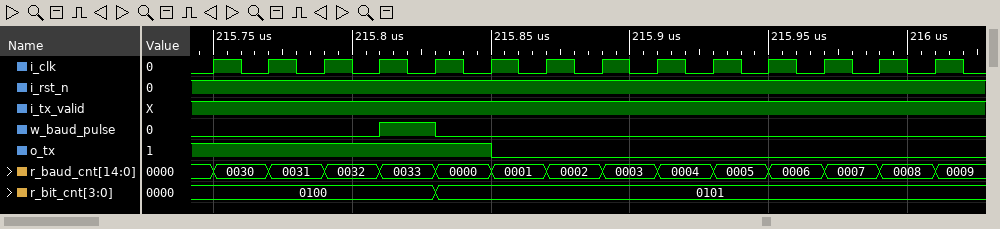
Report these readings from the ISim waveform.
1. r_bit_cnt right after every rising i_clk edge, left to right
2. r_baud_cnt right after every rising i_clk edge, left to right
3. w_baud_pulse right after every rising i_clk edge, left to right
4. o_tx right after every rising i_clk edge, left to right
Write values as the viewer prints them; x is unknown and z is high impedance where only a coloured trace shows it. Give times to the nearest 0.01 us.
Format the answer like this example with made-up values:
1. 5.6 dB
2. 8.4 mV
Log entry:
1. 0100, 0100, 0100, 0100, 0101, 0101, 0101, 0101, 0101, 0101, 0101, 0101, 0101, 0101
2. 0030, 0031, 0032, 0033, 0000, 0001, 0002, 0003, 0004, 0005, 0006, 0007, 0008, 0009
3. 0 0 0 1 0 0 0 0 0 0 0 0 0 0
4. 1 1 1 1 1 0 0 0 0 0 0 0 0 0
